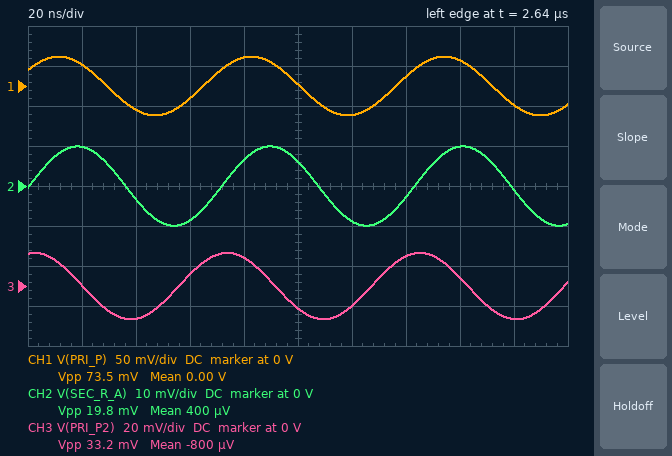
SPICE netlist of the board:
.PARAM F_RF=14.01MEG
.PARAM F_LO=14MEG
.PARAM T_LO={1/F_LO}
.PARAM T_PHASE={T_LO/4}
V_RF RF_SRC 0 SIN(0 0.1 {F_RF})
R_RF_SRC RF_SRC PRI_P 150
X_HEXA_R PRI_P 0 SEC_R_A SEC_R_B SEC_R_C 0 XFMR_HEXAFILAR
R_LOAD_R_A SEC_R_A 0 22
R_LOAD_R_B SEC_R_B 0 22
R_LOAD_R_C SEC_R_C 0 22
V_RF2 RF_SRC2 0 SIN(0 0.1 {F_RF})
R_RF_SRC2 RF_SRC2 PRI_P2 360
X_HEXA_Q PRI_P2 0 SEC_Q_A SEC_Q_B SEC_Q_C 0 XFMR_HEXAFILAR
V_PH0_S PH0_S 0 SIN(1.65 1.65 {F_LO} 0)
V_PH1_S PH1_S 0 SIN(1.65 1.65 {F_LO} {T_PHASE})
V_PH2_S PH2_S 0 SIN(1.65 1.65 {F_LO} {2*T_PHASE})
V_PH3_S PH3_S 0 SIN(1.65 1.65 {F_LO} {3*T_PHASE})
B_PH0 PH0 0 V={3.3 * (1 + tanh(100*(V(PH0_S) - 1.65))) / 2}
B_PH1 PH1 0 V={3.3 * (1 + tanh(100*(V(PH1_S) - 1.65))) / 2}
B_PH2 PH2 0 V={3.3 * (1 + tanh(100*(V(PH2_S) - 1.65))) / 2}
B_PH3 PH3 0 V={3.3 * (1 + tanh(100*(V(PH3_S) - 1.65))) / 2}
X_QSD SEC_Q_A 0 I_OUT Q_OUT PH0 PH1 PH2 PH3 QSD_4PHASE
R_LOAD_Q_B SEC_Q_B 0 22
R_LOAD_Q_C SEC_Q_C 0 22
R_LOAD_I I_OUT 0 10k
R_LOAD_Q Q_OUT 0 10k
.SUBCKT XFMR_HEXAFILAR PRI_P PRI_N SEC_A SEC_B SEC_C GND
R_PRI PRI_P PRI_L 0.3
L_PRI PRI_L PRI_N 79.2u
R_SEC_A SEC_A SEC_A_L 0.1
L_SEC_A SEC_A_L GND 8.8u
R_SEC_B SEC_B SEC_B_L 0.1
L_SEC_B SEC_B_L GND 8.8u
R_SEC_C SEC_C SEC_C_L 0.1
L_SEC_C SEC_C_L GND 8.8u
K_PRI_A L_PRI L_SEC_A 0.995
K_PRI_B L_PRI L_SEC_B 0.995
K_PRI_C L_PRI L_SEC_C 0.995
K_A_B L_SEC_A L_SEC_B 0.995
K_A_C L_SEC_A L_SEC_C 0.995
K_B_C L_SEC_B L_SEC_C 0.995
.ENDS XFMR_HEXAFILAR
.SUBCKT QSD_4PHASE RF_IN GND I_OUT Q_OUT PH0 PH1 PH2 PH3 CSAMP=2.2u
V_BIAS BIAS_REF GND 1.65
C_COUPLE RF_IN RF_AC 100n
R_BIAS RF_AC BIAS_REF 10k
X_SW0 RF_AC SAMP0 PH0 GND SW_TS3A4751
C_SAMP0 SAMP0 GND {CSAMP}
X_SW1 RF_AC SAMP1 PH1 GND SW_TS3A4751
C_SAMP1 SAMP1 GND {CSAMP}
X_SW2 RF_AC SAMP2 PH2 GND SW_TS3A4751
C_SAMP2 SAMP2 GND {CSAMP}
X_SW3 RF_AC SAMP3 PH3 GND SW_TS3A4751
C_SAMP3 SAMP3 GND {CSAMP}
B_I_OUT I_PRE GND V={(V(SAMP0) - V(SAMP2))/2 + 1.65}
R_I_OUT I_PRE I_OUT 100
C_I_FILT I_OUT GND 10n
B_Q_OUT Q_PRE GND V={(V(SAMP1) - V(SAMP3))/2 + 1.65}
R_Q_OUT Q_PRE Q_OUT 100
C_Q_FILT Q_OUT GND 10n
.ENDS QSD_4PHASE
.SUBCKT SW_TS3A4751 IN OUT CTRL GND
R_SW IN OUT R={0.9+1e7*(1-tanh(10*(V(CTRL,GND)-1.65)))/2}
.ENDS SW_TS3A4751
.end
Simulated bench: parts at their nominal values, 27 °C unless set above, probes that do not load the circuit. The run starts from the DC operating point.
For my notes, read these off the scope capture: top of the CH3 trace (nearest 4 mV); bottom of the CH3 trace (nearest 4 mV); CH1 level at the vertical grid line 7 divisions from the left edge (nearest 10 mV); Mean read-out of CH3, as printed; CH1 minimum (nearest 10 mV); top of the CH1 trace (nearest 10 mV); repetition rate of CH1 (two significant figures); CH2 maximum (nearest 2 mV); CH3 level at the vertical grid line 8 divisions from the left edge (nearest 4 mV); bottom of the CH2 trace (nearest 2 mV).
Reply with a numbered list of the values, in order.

1. 16 mV
2. -16 mV
3. 10 mV
4. -800 µV
5. -40 mV
6. 40 mV
7. 14 MHz
8. 10 mV
9. 4 mV
10. -10 mV
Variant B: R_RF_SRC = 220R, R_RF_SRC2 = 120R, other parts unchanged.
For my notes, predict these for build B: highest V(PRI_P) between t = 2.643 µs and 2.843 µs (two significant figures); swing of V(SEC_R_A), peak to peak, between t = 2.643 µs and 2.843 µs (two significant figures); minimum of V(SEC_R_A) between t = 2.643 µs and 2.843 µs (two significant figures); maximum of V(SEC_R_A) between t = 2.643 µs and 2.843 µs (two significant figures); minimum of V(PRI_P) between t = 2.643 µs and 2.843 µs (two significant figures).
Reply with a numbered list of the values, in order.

1. 28 mV
2. 15 mV
3. -7.6 mV
4. 7.6 mV
5. -28 mV
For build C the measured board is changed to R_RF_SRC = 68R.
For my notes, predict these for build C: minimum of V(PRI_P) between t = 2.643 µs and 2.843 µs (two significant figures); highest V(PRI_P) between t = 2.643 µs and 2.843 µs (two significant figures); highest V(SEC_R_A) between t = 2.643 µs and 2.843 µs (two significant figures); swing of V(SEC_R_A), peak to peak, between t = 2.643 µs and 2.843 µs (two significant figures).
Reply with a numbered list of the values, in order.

1. -57 mV
2. 57 mV
3. 15 mV
4. 31 mV
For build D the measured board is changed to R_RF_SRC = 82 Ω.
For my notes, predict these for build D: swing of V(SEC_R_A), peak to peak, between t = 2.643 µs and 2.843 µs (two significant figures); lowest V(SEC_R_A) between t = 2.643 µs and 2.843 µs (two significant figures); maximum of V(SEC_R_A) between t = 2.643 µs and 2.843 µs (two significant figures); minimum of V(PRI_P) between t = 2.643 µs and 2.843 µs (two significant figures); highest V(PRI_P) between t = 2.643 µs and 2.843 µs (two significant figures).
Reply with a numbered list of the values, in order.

1. 28 mV
2. -14 mV
3. 14 mV
4. -52 mV
5. 52 mV
